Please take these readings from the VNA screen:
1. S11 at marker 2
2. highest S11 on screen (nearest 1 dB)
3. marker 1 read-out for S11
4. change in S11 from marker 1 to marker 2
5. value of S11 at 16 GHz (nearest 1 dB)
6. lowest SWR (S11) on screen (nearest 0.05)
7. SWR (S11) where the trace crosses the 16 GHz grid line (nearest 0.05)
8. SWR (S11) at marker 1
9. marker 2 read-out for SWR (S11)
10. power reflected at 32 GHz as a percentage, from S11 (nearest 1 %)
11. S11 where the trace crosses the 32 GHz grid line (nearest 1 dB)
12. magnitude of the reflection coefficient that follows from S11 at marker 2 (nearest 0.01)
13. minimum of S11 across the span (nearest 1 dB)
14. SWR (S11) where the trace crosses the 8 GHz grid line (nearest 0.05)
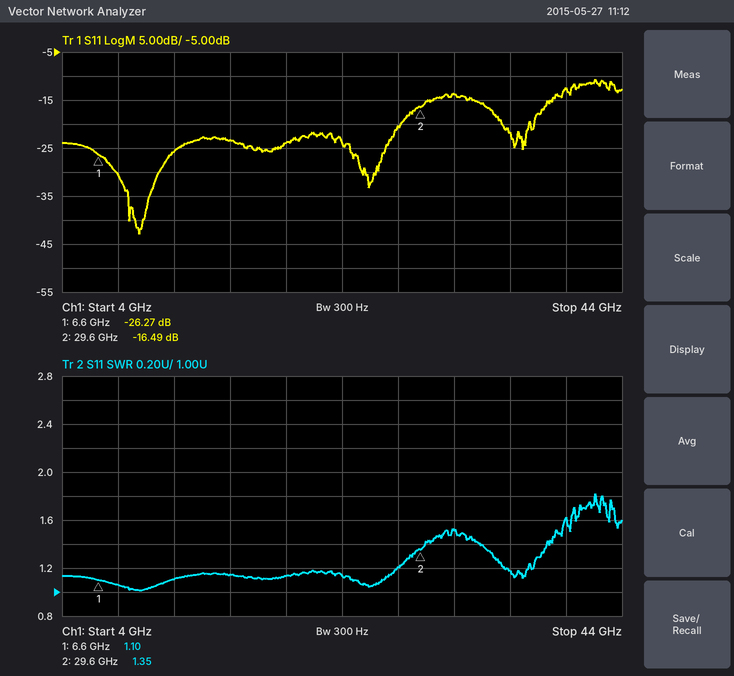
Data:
-16.49 dB
-11 dB
-26.27 dB
9.78 dB
-23 dB
1.00
1.15
1.10
1.35
4 %
-14 dB
0.15
-43 dB
1.05
